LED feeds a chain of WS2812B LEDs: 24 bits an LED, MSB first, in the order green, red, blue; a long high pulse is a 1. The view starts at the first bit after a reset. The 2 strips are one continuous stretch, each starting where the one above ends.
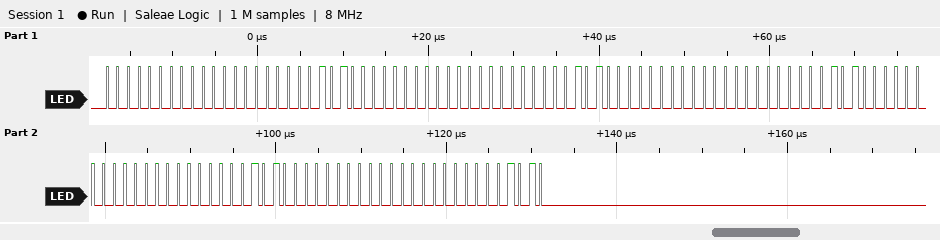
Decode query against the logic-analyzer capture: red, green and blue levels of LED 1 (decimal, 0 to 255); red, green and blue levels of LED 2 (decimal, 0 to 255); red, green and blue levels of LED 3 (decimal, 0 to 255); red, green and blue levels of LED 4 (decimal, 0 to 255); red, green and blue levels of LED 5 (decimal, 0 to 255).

0, 0, 10
0, 0, 10
0, 0, 10
0, 0, 10
0, 0, 10
